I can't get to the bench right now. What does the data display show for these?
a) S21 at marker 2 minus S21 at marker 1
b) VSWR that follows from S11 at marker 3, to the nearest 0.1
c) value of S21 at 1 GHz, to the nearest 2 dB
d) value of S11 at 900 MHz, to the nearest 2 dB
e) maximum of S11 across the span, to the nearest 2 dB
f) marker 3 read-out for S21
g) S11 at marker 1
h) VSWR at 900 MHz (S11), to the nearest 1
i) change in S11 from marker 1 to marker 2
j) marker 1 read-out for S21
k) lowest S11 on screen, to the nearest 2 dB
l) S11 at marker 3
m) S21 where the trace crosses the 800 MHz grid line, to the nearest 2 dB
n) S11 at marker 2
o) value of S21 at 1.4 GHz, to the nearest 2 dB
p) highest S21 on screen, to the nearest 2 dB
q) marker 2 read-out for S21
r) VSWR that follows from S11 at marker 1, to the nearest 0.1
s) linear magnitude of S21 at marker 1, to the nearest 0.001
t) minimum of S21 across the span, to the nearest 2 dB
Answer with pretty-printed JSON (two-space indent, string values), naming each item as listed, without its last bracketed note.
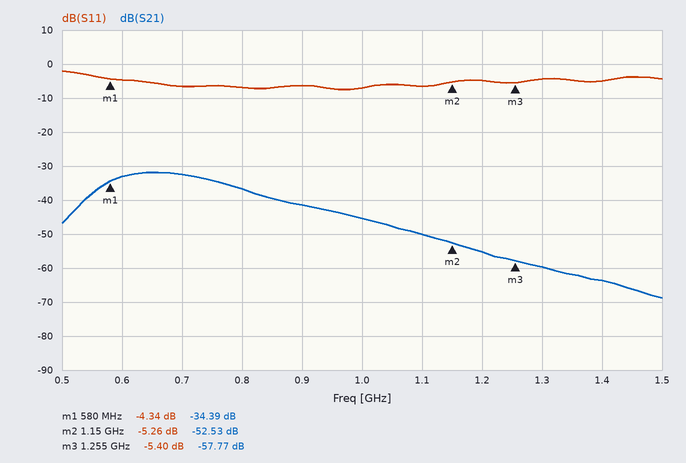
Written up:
{
  "S21 at marker 2 minus S21 at marker 1": "-18.14 dB",
  "VSWR that follows from S11 at marker 3, to the nearest 0.1": "3.3",
  "value of S21 at 1 GHz, to the nearest 2 dB": "-46 dB",
  "value of S11 at 900 MHz, to the nearest 2 dB": "-6 dB",
  "maximum of S11 across the span, to the nearest 2 dB": "-2 dB",
  "marker 3 read-out for S21": "-57.77 dB",
  "S11 at marker 1": "-4.34 dB",
  "VSWR at 900 MHz (S11), to the nearest 1": "3",
  "change in S11 from marker 1 to marker 2": "-0.92 dB",
  "marker 1 read-out for S21": "-34.39 dB",
  "lowest S11 on screen, to the nearest 2 dB": "-8 dB",
  "S11 at marker 3": "-5.40 dB",
  "S21 where the trace crosses the 800 MHz grid line, to the nearest 2 dB": "-36 dB",
  "S11 at marker 2": "-5.26 dB",
  "value of S21 at 1.4 GHz, to the nearest 2 dB": "-64 dB",
  "highest S21 on screen, to the nearest 2 dB": "-32 dB",
  "marker 2 read-out for S21": "-52.53 dB",
  "VSWR that follows from S11 at marker 1, to the nearest 0.1": "4.1",
  "linear magnitude of S21 at marker 1, to the nearest 0.001": "0.019",
  "minimum of S21 across the span, to the nearest 2 dB": "-68 dB"
}
